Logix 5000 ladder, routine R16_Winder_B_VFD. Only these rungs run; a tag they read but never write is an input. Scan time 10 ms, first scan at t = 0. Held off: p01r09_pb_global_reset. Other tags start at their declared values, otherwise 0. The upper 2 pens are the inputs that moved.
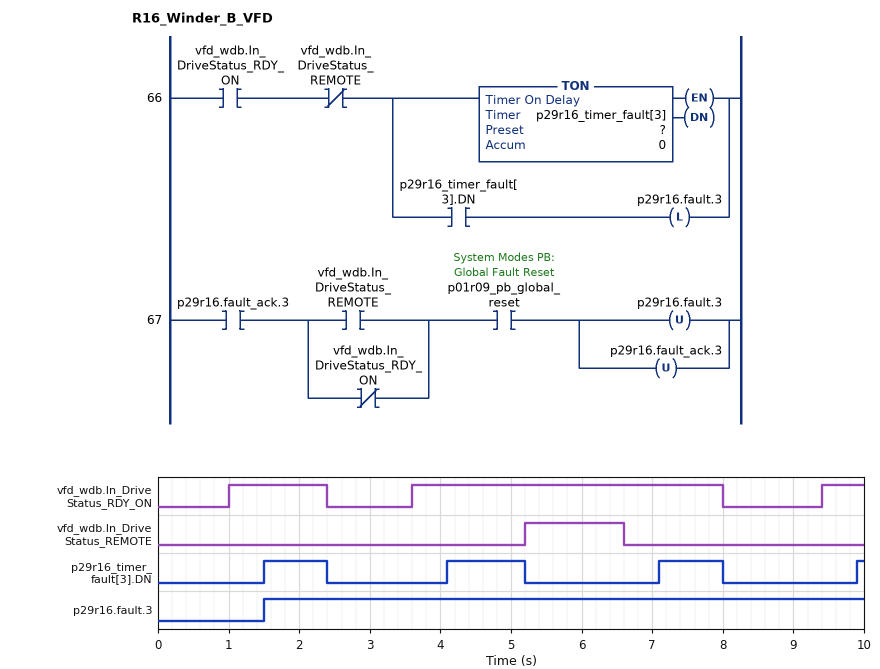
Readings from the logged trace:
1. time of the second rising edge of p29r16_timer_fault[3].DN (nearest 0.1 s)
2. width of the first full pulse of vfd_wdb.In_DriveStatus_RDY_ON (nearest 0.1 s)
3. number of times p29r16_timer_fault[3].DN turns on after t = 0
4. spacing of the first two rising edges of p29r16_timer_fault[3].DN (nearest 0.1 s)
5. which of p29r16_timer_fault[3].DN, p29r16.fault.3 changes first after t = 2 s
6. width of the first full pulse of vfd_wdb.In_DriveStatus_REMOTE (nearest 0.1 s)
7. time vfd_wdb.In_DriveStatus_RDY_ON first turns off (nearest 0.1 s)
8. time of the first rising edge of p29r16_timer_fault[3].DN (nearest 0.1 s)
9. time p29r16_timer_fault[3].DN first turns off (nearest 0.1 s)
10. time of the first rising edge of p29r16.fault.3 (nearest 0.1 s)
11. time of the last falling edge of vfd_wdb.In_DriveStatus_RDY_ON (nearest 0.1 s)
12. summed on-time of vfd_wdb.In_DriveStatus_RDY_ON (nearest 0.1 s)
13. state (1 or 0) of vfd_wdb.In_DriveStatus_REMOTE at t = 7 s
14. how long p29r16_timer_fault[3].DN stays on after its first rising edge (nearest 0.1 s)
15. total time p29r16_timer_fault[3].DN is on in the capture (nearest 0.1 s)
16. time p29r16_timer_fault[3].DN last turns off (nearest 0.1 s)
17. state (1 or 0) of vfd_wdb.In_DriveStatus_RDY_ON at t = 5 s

4.1 s
1.4 s
4
2.6 s
p29r16_timer_fault[3].DN
1.4 s
2.4 s
1.5 s
2.4 s
1.5 s
8.0 s
6.4 s
0
0.9 s
3.0 s
8.0 s
1
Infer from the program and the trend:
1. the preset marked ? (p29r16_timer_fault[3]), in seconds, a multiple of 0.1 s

0.5 s
